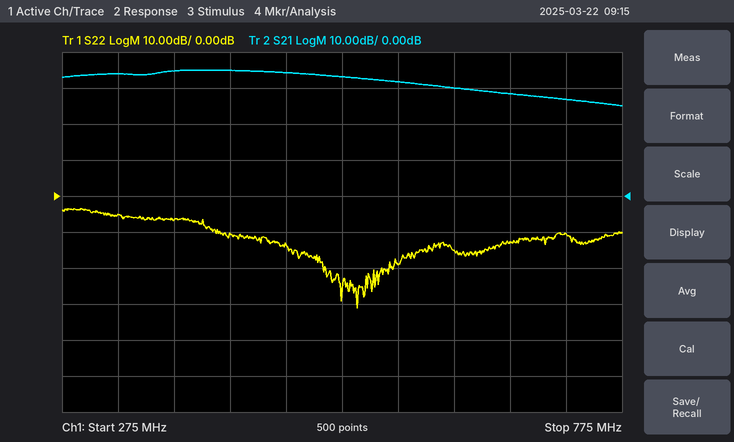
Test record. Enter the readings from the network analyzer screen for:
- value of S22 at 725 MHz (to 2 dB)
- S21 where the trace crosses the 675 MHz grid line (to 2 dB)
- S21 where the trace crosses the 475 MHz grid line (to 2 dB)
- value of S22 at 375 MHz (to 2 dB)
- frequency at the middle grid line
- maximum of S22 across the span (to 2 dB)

-10 dB
28 dB
34 dB
-6 dB
525 MHz
-4 dB
